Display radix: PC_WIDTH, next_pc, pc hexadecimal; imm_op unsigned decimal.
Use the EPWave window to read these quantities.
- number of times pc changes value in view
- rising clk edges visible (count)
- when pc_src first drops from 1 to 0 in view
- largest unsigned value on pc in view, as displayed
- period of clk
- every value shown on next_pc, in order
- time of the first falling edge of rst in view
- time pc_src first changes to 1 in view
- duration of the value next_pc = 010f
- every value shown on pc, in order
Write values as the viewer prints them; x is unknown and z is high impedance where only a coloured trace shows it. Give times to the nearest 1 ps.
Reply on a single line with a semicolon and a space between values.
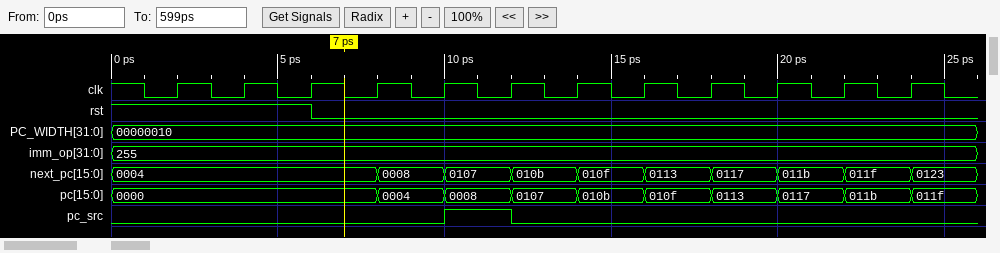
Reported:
9; 12; 12 ps; 011f; 2 ps; 0004, 0008, 0107, 010b, 010f, 0113, 0117, 011b, 011f, 0123; 6 ps; 10 ps; 2 ps; 0000, 0004, 0008, 0107, 010b, 010f, 0113, 0117, 011b, 011f
